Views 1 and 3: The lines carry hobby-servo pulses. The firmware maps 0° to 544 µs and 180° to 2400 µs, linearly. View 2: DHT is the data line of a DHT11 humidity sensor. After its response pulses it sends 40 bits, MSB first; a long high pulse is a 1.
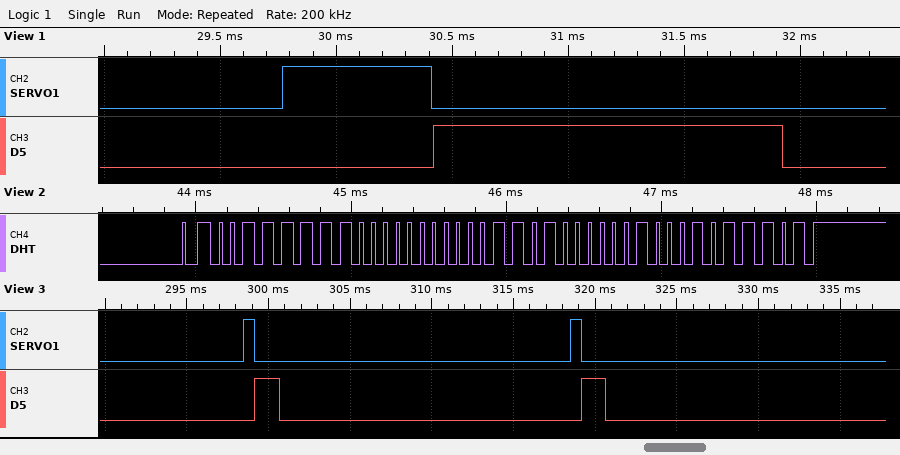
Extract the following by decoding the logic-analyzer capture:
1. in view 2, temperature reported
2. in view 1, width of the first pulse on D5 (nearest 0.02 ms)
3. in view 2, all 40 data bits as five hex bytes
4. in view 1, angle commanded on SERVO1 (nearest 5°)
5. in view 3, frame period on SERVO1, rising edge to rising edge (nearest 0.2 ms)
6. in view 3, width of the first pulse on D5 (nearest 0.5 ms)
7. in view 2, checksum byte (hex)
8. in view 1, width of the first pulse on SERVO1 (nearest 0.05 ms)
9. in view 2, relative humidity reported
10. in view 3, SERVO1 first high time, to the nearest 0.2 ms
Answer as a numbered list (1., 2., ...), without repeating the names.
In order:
1. 26.4 °C
2. 1.50 ms
3. 3F 00 1A 04 5D
4. 10°
5. 20.0 ms
6. 1.5 ms
7. 0x5D
8. 0.65 ms
9. 63 %
10. 0.6 ms
